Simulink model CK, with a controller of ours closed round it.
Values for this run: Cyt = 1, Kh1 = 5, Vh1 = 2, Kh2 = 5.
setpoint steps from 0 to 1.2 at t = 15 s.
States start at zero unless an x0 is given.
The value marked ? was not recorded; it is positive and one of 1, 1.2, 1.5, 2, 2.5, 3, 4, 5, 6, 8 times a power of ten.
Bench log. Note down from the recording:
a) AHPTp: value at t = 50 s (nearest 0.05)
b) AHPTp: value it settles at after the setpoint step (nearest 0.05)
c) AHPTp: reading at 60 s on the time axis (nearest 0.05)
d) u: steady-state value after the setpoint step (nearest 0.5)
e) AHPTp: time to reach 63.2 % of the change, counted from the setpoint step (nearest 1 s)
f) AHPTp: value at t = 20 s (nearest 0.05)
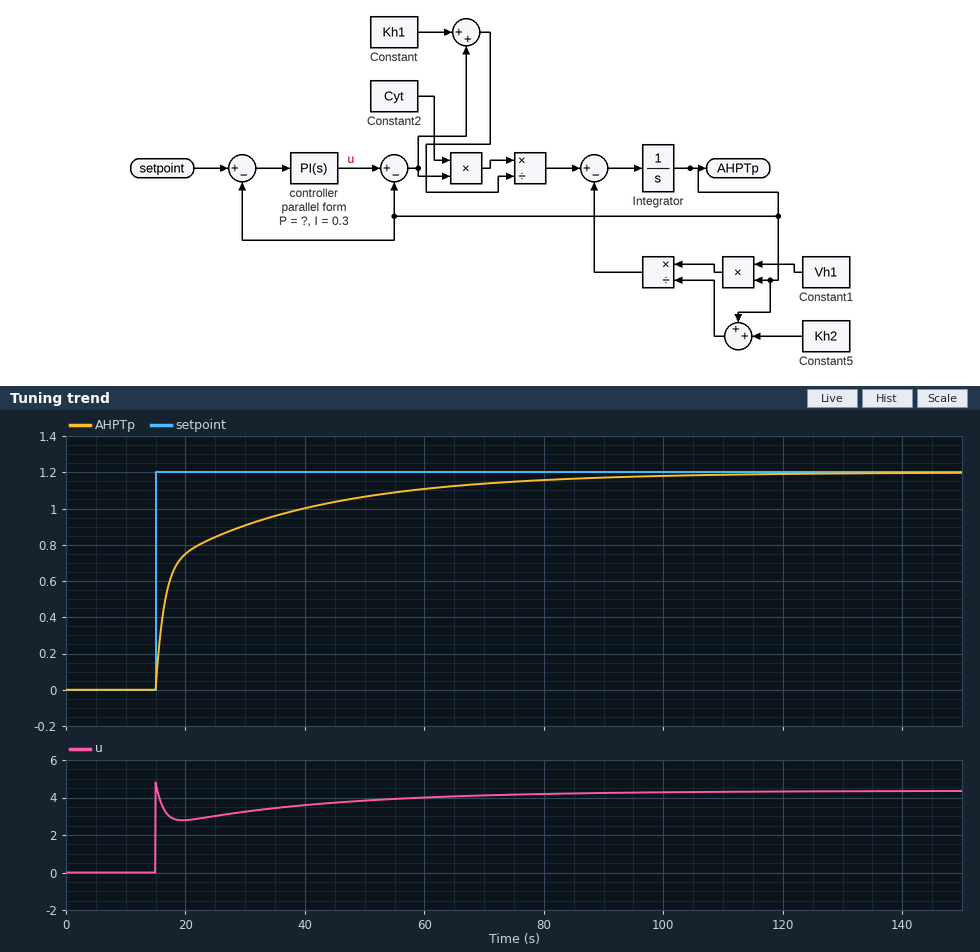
1.05
1.20
1.10
4.5
5 s
0.75
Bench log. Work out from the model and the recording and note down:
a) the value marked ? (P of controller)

4
